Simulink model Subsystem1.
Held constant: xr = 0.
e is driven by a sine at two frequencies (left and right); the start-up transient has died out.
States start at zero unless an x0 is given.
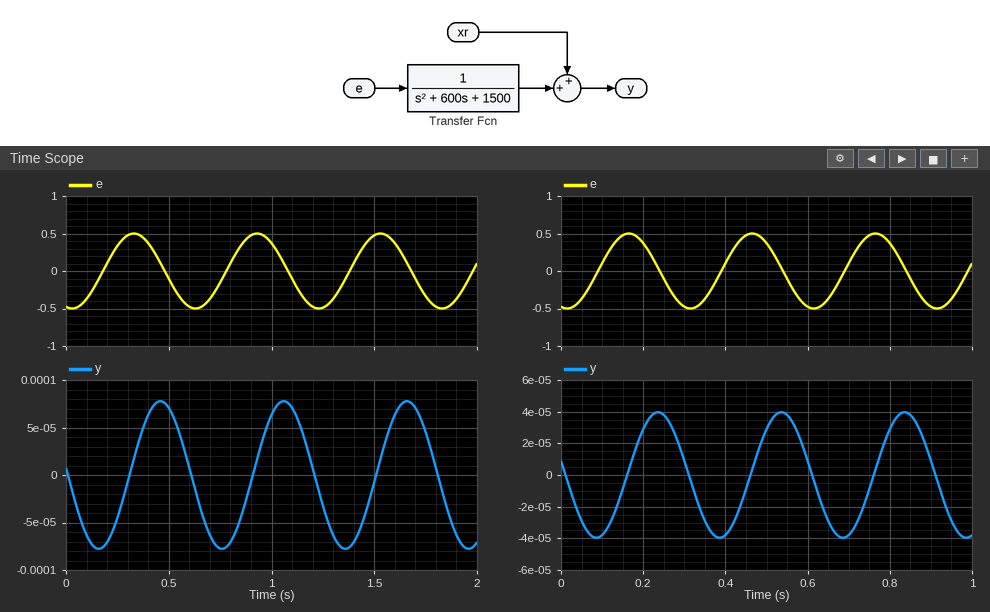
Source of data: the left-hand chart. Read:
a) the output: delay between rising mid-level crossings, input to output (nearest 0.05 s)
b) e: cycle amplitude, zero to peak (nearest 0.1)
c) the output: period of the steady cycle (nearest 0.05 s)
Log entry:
0.15 s
0.5
0.60 s
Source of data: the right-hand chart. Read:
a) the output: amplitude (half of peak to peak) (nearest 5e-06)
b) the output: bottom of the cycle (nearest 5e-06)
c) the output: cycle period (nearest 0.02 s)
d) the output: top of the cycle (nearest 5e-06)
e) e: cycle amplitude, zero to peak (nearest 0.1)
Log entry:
0.000040
-0.000040
0.30 s
0.000040
0.5
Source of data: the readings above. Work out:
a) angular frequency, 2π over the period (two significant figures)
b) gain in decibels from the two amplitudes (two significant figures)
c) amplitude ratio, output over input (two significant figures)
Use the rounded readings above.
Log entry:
21 rad/s
-82 dB
0.000080
